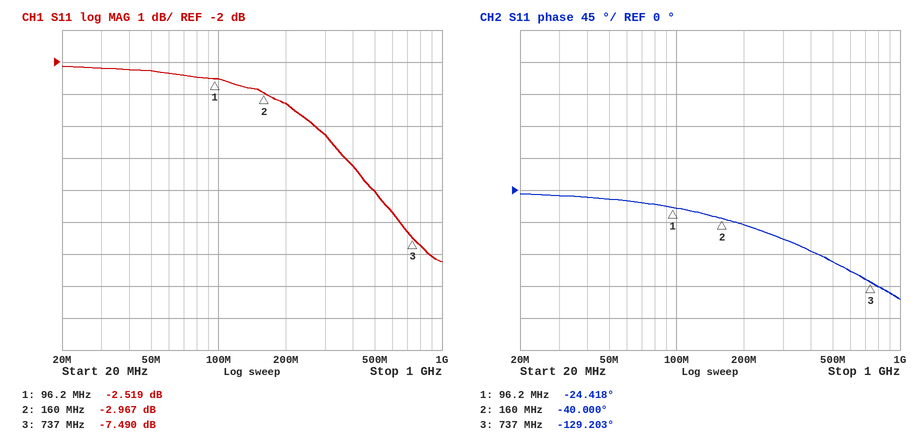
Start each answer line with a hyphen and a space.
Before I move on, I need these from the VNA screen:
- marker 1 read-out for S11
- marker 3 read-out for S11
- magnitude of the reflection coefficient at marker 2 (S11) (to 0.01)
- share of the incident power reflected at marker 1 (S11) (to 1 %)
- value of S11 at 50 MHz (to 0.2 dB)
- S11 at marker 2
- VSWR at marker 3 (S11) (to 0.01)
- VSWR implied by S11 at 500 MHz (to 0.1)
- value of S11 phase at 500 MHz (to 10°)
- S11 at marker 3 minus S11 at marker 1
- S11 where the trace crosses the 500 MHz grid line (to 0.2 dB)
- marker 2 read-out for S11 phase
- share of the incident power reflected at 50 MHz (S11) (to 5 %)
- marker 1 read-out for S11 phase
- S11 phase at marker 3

- -2.519 dB
- -7.490 dB
- 0.71
- 56 %
- -2.2 dB
- -2.967 dB
- 2.46
- 3.0
- -100°
- -4.971 dB
- -6.0 dB
- -40.000°
- 60 %
- -24.418°
- -129.203°
